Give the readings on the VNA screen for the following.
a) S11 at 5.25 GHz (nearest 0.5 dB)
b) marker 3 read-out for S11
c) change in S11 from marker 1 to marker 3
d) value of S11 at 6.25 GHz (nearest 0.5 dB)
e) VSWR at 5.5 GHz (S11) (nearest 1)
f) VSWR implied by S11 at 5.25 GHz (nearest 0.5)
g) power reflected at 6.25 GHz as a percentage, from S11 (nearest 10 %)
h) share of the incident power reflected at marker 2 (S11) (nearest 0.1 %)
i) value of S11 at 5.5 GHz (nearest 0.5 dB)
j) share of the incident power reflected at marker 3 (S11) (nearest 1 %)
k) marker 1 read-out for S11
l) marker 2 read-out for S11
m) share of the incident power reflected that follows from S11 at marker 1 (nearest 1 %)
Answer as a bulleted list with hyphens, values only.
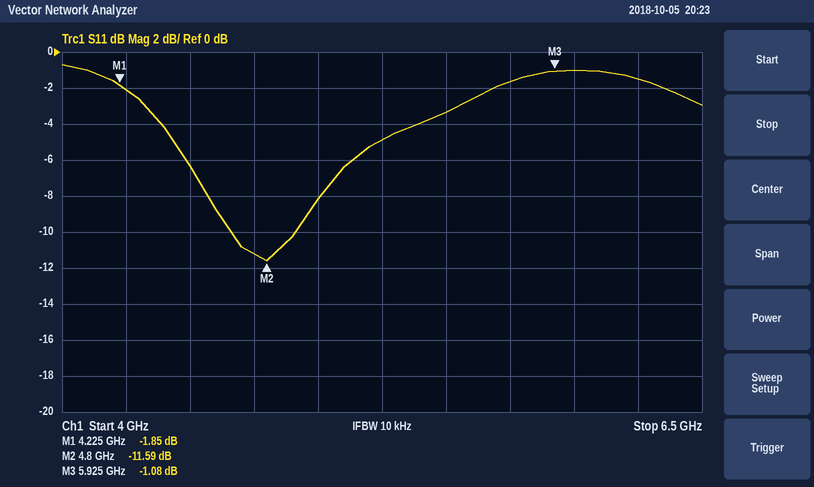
- -5.0 dB
- -1.08 dB
- 0.77 dB
- -1.5 dB
- 5
- 3.5
- 70 %
- 6.9 %
- -3.5 dB
- 78 %
- -1.85 dB
- -11.59 dB
- 65 %
